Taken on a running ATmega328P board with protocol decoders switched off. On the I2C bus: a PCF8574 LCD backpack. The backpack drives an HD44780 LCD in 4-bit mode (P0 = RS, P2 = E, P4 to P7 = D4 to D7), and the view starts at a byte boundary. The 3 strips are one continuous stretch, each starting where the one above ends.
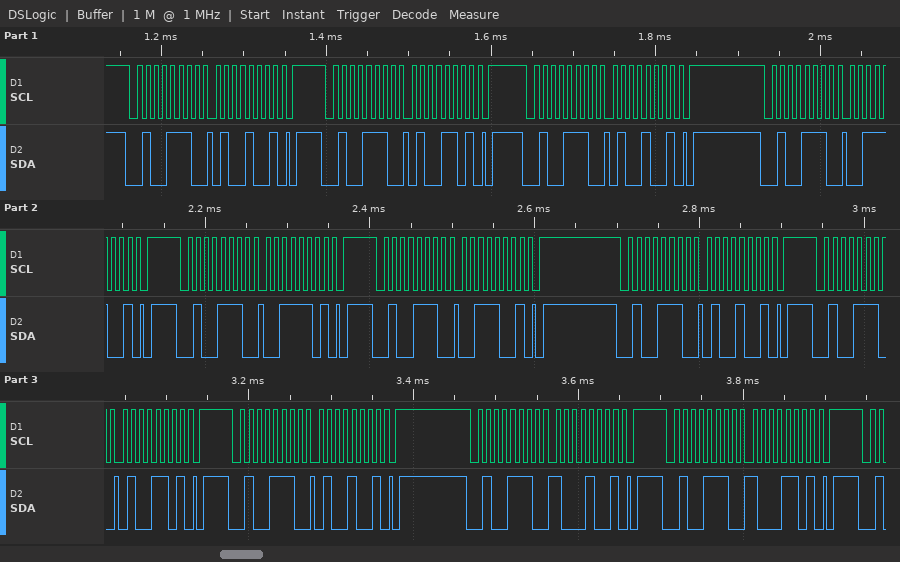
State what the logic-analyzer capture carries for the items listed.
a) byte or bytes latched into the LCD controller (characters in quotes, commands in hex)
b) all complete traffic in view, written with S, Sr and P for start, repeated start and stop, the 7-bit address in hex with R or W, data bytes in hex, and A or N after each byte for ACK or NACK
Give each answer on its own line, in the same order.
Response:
'C'
S 27W A 49 A P S 27W A 4D A P S 27W A 49 A P S 27W A 39 A P S 27W A 3D A P S 27W A 39 A P S 27W A 49 A P S 27W A 4D A P S 27W A 49 A P S 27W A 89 A P S 27W A 8D A P
